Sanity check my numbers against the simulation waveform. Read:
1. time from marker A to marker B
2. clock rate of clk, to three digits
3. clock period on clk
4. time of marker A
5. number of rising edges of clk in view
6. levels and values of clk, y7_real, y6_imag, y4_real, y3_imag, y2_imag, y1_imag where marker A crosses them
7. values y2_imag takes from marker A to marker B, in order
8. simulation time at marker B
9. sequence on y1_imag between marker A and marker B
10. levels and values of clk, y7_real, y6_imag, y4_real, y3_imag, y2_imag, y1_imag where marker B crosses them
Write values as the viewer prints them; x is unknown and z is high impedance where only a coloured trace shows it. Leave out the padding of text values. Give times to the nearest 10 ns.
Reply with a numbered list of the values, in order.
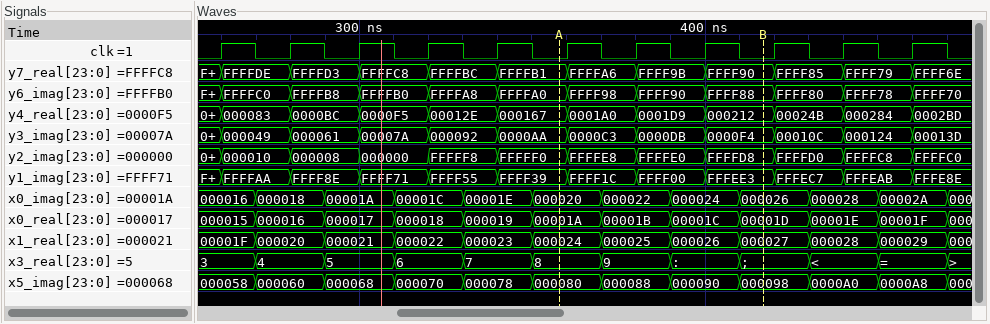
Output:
1. 60 ns
2. 50.0 MHz
3. 20 ns
4. 360 ns
5. 11
6. clk=0, y7_real=FFFFB1, y6_imag=FFFFA0, y4_real=000167, y3_imag=0000AA, y2_imag=FFFFF0, y1_imag=FFFF39
7. FFFFF0, FFFFE8, FFFFE0, FFFFD8
8. 420 ns
9. FFFF39, FFFF1C, FFFF00, FFFEE3
10. clk=0, y7_real=FFFF90, y6_imag=FFFF88, y4_real=000212, y3_imag=0000F4, y2_imag=FFFFD8, y1_imag=FFFEE3
